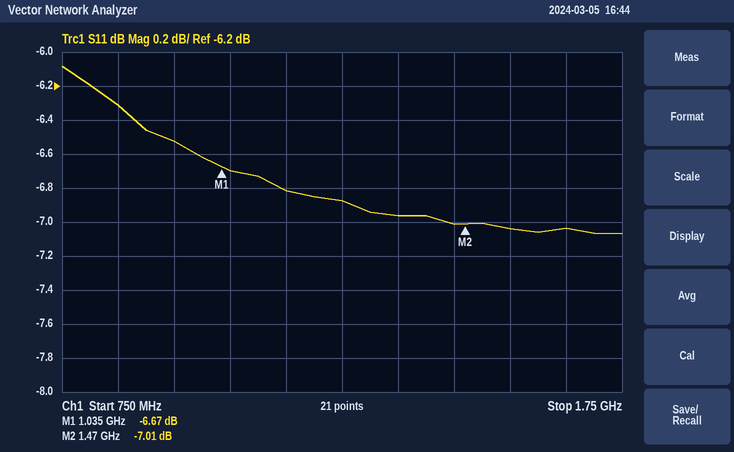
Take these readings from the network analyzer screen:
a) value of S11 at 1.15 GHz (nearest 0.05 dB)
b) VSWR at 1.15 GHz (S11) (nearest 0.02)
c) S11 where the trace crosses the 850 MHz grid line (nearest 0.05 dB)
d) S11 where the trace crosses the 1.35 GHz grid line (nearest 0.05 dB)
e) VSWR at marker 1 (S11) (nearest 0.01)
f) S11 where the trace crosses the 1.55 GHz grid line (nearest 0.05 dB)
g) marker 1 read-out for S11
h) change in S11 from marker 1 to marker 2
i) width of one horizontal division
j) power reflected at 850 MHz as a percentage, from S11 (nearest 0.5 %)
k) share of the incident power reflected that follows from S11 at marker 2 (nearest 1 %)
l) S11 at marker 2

-6.80 dB
2.68
-6.30 dB
-6.95 dB
2.73
-7.05 dB
-6.67 dB
-0.34 dB
100 MHz
23.5 %
20 %
-7.01 dB
